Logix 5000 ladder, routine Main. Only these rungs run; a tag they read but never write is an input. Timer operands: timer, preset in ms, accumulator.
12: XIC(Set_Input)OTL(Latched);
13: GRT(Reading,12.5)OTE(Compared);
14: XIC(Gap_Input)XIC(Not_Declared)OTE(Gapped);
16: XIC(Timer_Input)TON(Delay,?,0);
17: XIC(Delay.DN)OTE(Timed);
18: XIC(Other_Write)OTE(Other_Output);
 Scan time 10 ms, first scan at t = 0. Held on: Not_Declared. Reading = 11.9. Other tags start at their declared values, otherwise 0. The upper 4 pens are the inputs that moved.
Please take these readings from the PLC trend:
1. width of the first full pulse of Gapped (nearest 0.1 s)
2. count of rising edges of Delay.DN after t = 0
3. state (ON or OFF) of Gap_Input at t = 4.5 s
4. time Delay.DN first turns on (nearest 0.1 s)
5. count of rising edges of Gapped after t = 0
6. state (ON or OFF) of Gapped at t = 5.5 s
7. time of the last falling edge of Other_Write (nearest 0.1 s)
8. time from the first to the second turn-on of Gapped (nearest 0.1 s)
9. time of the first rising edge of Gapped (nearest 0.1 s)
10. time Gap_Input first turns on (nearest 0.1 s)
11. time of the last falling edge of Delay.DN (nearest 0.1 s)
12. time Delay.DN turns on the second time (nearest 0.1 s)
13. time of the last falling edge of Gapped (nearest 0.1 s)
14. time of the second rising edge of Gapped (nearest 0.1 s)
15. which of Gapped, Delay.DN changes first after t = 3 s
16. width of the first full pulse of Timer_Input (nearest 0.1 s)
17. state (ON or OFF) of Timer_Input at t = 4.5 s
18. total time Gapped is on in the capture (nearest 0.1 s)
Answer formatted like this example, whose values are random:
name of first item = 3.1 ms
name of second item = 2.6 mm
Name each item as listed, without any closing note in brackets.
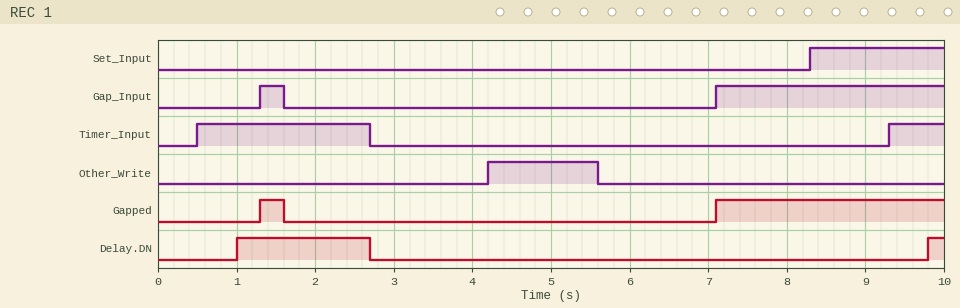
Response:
width of the first full pulse of Gapped = 0.3 s
count of rising edges of Delay.DN after t = 0 = 2
state (ON or OFF) of Gap_Input at t = 4.5 s = OFF
time Delay.DN first turns on = 1.0 s
count of rising edges of Gapped after t = 0 = 2
state (ON or OFF) of Gapped at t = 5.5 s = OFF
time of the last falling edge of Other_Write = 5.6 s
time from the first to the second turn-on of Gapped = 5.8 s
time of the first rising edge of Gapped = 1.3 s
time Gap_Input first turns on = 1.3 s
time of the last falling edge of Delay.DN = 2.7 s
time Delay.DN turns on the second time = 9.8 s
time of the last falling edge of Gapped = 1.6 s
time of the second rising edge of Gapped = 7.1 s
which of Gapped, Delay.DN changes first after t = 3 s = Gapped
width of the first full pulse of Timer_Input = 2.2 s
state (ON or OFF) of Timer_Input at t = 4.5 s = OFF
total time Gapped is on in the capture = 3.2 s
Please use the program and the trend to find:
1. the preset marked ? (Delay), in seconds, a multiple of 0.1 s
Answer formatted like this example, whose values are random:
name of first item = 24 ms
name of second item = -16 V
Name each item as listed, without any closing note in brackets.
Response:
the preset marked ? (Delay), in seconds, a multiple of 0.1 s = 0.5 s
